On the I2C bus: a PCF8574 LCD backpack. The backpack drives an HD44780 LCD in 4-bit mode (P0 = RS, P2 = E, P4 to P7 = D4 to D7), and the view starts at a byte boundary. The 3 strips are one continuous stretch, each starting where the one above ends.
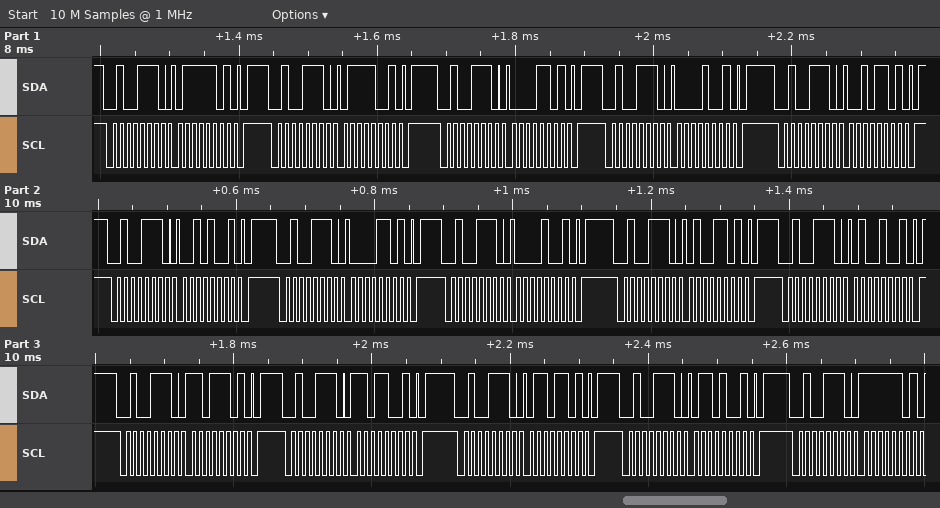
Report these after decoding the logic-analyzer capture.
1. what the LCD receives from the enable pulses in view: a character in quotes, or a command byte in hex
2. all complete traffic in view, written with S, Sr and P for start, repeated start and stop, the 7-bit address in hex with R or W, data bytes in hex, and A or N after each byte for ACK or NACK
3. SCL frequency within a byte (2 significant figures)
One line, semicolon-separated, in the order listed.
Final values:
'p' ' ' 'M'; S 27W A 7D A P S 27W A 79 A P S 27W A 0D A P S 27W A 09 A P S 27W A 2D A P S 27W A 29 A P S 27W A 0D A P S 27W A 09 A P S 27W A 4D A P S 27W A 49 A P S 27W A DD A P S 27W A D9 A P S 27W A 6D A P S 27W A 69 A P S 27W A FD A; 100 kHz
